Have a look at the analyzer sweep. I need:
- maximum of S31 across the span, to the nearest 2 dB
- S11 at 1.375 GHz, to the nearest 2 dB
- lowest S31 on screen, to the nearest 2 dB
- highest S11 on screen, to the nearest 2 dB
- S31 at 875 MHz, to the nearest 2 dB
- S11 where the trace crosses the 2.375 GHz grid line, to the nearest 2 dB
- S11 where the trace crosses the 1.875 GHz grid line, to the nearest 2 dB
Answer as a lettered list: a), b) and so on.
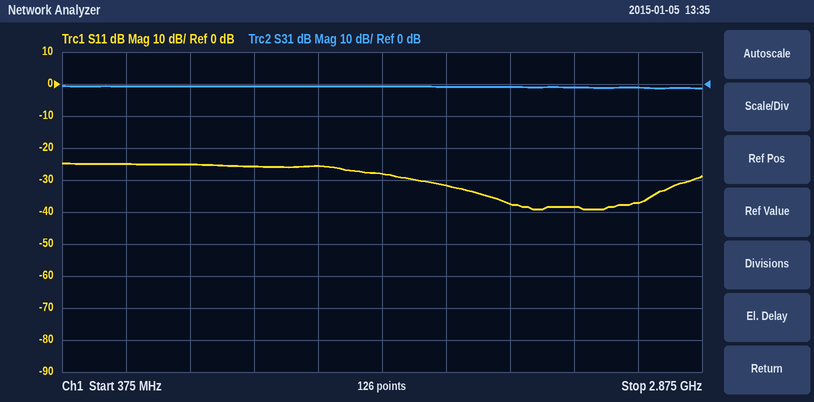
a) 0 dB
b) -26 dB
c) -2 dB
d) -24 dB
e) 0 dB
f) -38 dB
g) -32 dB
